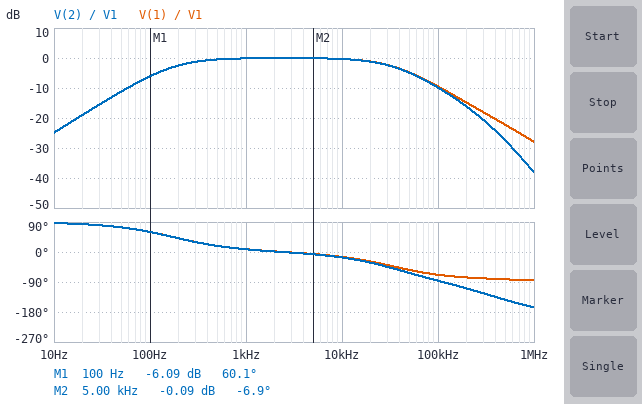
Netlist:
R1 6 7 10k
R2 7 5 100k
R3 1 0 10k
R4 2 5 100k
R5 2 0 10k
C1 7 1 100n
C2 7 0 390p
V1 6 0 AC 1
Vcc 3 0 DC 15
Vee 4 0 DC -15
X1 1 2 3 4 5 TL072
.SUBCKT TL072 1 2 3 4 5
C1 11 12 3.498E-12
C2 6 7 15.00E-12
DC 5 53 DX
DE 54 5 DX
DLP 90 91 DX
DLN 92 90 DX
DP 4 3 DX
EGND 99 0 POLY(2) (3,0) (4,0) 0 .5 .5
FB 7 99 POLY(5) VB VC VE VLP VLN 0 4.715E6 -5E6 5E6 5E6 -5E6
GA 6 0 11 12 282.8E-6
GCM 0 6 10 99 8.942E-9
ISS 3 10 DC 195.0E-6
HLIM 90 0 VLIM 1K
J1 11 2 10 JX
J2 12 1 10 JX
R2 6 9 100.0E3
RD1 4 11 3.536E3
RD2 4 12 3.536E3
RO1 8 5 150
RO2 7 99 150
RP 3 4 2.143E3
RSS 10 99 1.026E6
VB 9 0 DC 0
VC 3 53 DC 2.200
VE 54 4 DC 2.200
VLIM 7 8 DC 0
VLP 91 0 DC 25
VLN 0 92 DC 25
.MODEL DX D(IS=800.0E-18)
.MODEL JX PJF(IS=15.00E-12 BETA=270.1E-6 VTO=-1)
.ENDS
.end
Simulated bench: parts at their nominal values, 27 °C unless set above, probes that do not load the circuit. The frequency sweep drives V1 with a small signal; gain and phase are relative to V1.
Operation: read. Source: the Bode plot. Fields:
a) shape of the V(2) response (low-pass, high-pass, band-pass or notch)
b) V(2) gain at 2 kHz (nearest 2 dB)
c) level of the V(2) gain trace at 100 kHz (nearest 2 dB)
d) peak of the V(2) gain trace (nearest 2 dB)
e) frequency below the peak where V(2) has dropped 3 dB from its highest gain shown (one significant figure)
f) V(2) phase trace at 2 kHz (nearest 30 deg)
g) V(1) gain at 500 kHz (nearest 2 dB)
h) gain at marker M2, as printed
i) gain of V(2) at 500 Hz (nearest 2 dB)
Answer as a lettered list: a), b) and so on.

a) band-pass
b) 0 dB
c) -10 dB
d) 0 dB
e) 200 Hz
f) 0 deg
g) -22 dB
h) -0.09 dB
i) 0 dB
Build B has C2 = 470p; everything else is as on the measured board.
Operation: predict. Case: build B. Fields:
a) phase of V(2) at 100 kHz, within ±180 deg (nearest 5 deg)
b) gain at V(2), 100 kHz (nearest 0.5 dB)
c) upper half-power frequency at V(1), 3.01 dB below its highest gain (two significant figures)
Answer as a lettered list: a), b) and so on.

a) -90 deg
b) -11.0 dB
c) 30 kHz
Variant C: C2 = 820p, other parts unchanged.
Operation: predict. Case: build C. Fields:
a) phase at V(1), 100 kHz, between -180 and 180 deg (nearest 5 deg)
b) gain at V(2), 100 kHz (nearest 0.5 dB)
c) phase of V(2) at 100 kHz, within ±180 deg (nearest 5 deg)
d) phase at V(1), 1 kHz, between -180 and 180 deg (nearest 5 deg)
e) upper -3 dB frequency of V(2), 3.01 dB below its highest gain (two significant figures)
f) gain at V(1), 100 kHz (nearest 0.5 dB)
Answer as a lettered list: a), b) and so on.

a) -80 deg
b) -15.5 dB
c) -95 deg
d) 5 deg
e) 18 kHz
f) -15.0 dB
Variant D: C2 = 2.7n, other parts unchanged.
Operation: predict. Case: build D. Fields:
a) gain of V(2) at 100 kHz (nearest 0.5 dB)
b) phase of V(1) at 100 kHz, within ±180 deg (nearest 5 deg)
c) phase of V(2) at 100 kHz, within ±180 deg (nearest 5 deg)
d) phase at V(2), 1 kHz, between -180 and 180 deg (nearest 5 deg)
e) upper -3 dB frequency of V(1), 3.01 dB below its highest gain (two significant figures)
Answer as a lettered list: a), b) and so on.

a) -25.0 dB
b) -85 deg
c) -105 deg
d) 0 deg
e) 6.1 kHz
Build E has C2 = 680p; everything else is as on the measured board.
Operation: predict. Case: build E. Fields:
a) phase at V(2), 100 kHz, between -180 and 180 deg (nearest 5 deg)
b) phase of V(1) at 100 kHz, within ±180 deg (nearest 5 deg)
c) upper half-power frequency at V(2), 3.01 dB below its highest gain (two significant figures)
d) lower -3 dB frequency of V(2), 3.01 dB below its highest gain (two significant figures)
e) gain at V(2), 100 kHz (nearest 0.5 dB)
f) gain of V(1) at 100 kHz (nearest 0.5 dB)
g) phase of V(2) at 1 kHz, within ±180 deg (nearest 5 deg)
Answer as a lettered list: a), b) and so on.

a) -95 deg
b) -75 deg
c) 22 kHz
d) 170 Hz
e) -14.0 dB
f) -13.5 dB
g) 5 deg
